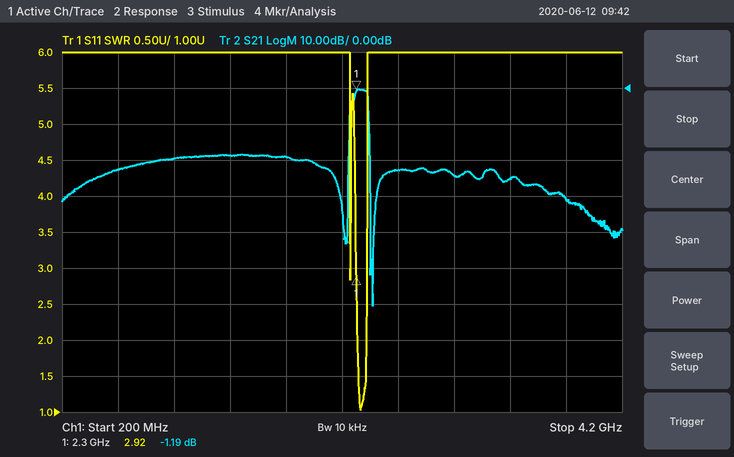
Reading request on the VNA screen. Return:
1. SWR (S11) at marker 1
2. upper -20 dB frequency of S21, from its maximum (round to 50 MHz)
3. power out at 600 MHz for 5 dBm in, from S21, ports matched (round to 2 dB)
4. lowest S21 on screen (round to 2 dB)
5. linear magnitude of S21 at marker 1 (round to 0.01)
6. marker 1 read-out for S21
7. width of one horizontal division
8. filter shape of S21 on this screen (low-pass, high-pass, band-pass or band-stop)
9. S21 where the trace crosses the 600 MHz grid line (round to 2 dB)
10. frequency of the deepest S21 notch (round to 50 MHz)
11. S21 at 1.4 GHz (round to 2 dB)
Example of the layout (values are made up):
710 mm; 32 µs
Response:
2.92; 2.40 GHz; -18 dBm; -60 dB; 0.87; -1.19 dB; 400 MHz; band-pass; -22 dB; 2.40 GHz; -18 dB
